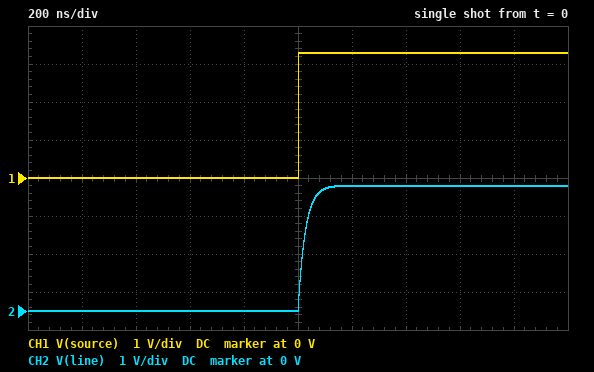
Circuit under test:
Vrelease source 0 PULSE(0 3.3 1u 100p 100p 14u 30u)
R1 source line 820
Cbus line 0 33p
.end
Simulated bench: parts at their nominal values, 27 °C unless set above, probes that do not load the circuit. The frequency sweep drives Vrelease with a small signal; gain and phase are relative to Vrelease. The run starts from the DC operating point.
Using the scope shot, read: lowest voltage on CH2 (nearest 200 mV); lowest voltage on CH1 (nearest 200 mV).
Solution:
0 V
0 V
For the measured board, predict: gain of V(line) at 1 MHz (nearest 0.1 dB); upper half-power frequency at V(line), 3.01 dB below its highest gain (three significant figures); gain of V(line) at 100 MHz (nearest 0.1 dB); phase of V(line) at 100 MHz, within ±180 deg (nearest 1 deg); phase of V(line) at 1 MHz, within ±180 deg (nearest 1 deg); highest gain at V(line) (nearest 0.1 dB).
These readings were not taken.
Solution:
-0.1 dB
5.88 MHz
-24.6 dB
-87 deg
-10 deg
0 dB
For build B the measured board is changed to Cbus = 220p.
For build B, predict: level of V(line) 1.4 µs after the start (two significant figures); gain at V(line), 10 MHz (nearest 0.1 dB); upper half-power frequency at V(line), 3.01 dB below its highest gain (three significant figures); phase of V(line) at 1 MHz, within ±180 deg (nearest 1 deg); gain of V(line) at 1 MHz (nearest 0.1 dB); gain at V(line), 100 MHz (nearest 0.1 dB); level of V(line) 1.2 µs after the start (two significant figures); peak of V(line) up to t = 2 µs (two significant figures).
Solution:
2.9 V
-21.1 dB
882 kHz
-49 deg
-3.6 dB
-41.1 dB
2.2 V
3.3 V
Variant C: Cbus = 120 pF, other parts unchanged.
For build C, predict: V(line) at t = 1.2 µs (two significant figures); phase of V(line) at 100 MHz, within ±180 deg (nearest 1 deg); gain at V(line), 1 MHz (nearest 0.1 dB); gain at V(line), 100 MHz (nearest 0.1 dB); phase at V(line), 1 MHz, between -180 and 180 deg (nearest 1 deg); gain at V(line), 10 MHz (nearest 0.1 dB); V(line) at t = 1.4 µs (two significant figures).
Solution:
2.9 V
-89 deg
-1.4 dB
-35.8 dB
-32 deg
-15.9 dB
3.2 V
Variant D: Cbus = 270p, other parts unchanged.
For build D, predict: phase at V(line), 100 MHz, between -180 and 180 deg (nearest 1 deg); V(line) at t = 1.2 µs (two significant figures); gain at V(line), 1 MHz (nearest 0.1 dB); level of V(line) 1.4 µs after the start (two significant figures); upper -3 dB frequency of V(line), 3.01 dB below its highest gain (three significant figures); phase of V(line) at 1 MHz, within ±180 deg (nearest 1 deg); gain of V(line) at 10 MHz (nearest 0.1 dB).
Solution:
-90 deg
2.0 V
-4.7 dB
2.8 V
719 kHz
-54 deg
-22.9 dB
